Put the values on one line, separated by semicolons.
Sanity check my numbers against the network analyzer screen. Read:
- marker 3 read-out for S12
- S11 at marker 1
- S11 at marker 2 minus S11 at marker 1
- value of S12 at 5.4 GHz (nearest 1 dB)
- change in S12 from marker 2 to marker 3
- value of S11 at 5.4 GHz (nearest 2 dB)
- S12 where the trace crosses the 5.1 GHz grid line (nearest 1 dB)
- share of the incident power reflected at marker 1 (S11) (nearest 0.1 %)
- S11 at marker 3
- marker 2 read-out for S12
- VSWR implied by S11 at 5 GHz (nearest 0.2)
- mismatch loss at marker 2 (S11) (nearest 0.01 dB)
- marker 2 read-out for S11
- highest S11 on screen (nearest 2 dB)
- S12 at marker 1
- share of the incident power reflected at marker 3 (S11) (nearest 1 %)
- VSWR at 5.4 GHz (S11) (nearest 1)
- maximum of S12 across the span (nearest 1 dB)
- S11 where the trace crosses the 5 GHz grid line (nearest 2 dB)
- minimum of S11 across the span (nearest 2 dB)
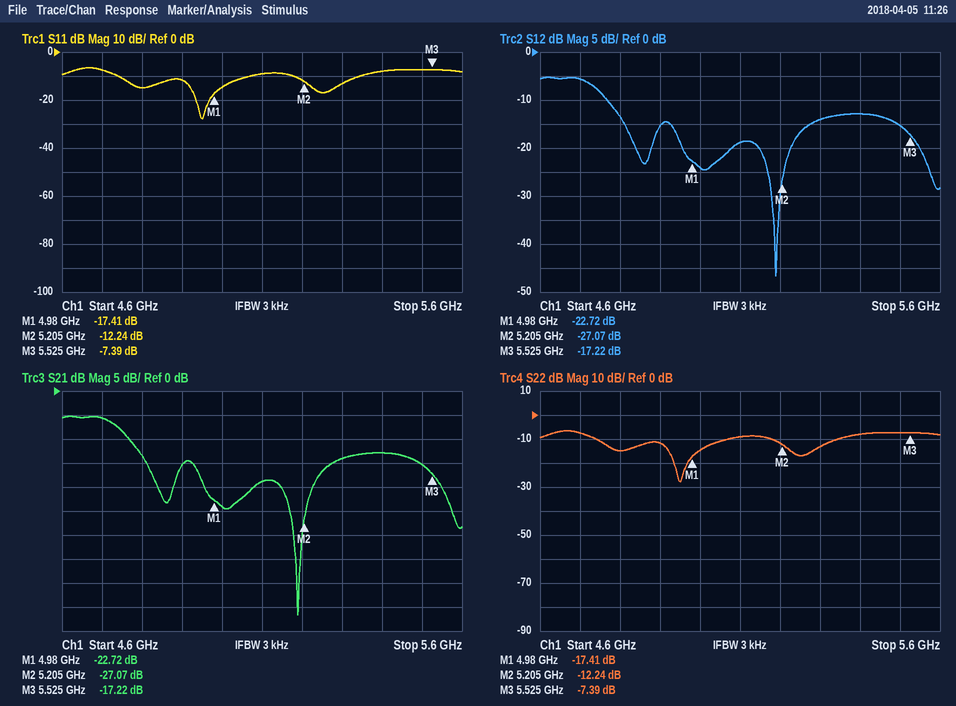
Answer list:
-17.22 dB; -17.41 dB; 5.17 dB; -13 dB; 9.85 dB; -8 dB; -19 dB; 1.8 %; -7.39 dB; -27.07 dB; 1.4; 0.27 dB; -12.24 dB; -6 dB; -22.72 dB; 18 %; 2; -5 dB; -14 dB; -28 dB
